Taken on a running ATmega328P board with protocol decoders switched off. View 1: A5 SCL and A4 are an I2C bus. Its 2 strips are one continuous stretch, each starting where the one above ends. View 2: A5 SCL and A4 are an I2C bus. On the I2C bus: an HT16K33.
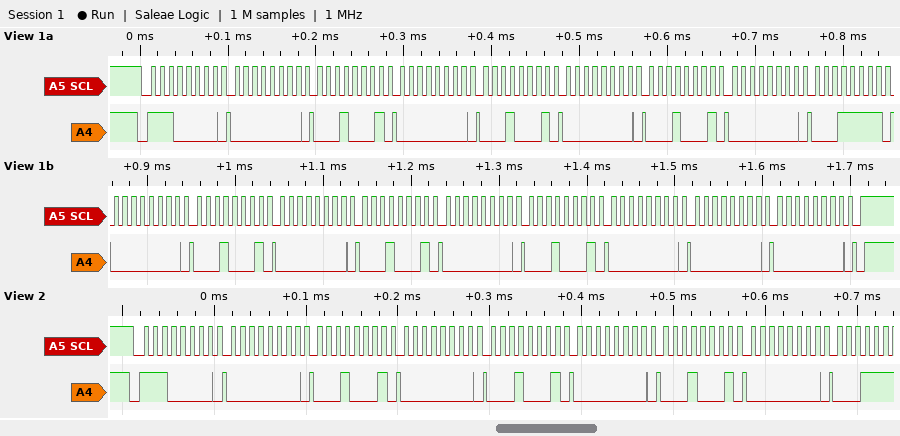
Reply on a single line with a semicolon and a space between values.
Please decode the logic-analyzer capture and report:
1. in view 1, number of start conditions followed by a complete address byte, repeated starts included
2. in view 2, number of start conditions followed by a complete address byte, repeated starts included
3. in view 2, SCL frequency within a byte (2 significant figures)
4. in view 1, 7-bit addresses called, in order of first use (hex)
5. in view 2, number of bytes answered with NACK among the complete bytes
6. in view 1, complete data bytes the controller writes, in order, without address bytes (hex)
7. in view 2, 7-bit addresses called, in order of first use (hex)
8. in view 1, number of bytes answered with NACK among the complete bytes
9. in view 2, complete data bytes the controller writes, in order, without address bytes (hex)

1; 1; 100 kHz; 0x70; 0; 00 11 00 11 00 11 00 1F 00 11 00 11 00 11 00 00 00; 0x70; 0; 00 11 00 11 00 11 00
